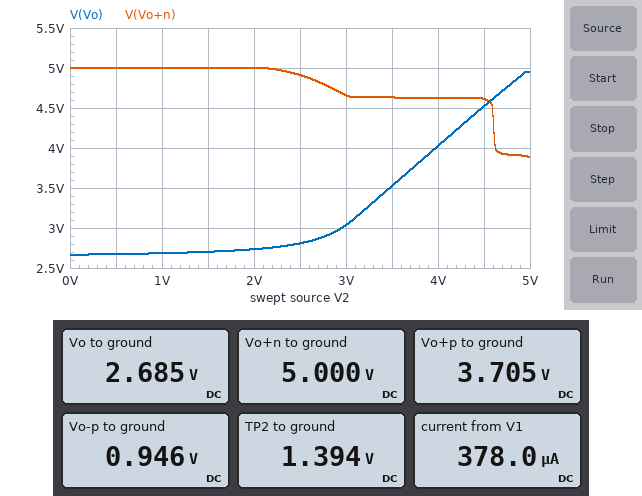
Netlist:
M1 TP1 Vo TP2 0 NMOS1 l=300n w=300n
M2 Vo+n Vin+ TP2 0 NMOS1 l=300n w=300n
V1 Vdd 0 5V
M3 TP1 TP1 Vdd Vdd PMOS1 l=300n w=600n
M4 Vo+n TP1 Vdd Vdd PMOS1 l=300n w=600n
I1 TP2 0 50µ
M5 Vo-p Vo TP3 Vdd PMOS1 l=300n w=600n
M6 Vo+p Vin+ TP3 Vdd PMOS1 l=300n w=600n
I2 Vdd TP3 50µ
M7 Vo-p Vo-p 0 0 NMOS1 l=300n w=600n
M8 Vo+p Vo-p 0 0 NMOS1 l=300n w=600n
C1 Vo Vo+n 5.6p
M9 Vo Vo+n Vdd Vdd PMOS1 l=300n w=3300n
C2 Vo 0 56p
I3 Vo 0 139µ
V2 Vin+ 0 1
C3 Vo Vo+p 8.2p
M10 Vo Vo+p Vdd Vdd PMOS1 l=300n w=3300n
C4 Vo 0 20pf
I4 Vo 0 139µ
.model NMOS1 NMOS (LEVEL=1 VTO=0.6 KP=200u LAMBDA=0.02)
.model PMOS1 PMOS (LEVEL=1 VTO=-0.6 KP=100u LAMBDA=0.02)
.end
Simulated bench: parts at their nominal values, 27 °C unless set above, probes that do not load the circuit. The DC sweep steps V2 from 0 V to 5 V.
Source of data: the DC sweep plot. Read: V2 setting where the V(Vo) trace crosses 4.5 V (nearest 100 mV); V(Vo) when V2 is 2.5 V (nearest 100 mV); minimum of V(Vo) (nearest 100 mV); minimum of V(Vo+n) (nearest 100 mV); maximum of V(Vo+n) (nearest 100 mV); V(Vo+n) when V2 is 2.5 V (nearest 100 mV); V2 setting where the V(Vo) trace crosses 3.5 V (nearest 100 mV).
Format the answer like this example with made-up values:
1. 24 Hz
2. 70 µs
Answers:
1. 4.5 V
2. 2.8 V
3. 2.7 V
4. 3.9 V
5. 5.0 V
6. 4.9 V
7. 3.5 V
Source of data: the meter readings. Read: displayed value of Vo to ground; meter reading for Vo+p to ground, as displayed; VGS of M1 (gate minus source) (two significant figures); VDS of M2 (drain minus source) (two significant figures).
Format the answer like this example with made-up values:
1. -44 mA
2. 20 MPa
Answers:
1. 2.685 V
2. 3.705 V
3. 1.3 V
4. 3.6 V
